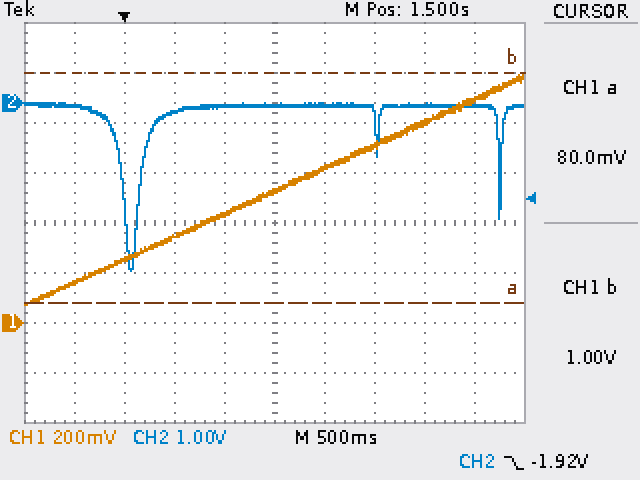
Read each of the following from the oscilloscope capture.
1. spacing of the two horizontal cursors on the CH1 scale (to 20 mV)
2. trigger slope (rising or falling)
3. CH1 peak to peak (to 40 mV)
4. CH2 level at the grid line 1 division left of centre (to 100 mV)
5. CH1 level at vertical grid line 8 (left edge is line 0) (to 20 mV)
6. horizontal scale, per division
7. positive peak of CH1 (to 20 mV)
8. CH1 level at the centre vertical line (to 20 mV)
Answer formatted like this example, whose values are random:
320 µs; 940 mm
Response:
920 mV; falling; 920 mV; -100 mV; 800 mV; 500 ms; 1.00 V; 520 mV
